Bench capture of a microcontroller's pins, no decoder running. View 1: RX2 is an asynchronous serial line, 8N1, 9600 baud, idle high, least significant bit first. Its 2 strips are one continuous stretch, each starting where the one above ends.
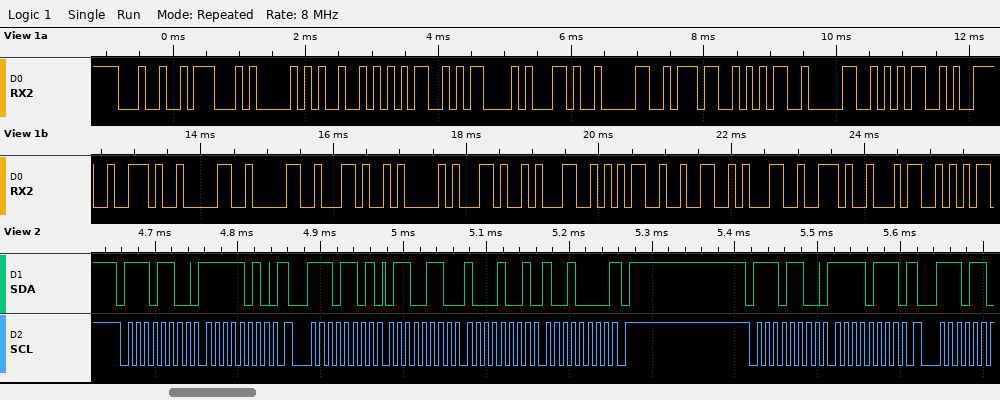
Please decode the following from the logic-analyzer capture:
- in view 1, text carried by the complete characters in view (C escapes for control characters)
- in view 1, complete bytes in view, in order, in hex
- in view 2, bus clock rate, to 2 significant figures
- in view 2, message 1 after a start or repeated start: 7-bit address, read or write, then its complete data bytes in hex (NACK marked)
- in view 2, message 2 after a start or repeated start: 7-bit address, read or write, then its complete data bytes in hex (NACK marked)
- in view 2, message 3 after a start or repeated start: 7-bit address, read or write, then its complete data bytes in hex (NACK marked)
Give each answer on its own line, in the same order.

"$GPRMC,075059.00,A,1521.4"
24 47 50 52 4D 43 2C 30 37 35 30 35 39 2E 30 30 2C 41 2C 31 35 32 31 2E 34
100 kHz
0x76 write: FA
0x76 read: 66 89 90 NACK
0x76 write: F7
